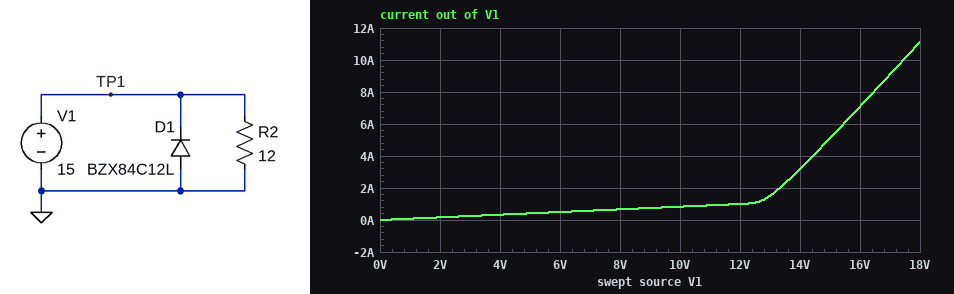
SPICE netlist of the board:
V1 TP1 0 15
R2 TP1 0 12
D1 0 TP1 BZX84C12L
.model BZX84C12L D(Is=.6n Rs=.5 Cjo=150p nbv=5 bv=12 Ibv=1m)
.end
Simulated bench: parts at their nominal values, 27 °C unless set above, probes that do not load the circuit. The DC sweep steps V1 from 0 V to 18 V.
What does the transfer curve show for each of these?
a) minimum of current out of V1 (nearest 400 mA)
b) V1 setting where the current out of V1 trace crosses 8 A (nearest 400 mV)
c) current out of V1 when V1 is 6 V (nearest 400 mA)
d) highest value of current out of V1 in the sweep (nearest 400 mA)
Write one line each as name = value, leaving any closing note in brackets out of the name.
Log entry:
minimum of current out of V1 = 0 A
V1 setting where the current out of V1 trace crosses 8 A = 16.4 V
current out of V1 when V1 is 6 V = 400 mA
highest value of current out of V1 in the sweep = 11.2 A
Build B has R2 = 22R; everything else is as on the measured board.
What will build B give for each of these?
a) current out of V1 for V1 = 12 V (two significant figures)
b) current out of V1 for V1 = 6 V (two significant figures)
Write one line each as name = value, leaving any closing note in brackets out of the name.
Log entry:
current out of V1 for V1 = 12 V = 550 mA
current out of V1 for V1 = 6 V = 270 mA
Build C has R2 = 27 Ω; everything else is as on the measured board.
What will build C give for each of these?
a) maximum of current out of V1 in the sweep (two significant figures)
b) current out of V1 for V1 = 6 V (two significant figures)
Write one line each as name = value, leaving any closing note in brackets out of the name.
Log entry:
maximum of current out of V1 in the sweep = 10 A
current out of V1 for V1 = 6 V = 220 mA
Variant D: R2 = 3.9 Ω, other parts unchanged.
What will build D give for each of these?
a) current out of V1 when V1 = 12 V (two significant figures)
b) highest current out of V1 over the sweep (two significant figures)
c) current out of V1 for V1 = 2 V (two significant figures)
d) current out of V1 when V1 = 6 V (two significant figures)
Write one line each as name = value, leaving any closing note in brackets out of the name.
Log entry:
current out of V1 when V1 = 12 V = 3.1 A
highest current out of V1 over the sweep = 14 A
current out of V1 for V1 = 2 V = 510 mA
current out of V1 when V1 = 6 V = 1.5 A
